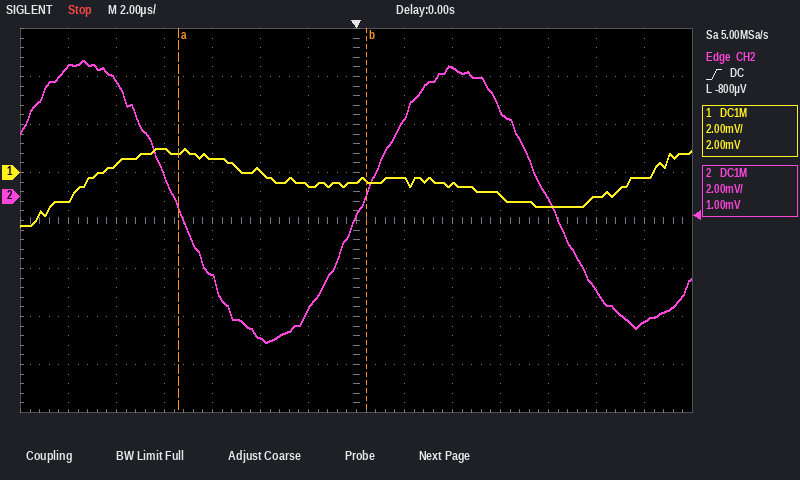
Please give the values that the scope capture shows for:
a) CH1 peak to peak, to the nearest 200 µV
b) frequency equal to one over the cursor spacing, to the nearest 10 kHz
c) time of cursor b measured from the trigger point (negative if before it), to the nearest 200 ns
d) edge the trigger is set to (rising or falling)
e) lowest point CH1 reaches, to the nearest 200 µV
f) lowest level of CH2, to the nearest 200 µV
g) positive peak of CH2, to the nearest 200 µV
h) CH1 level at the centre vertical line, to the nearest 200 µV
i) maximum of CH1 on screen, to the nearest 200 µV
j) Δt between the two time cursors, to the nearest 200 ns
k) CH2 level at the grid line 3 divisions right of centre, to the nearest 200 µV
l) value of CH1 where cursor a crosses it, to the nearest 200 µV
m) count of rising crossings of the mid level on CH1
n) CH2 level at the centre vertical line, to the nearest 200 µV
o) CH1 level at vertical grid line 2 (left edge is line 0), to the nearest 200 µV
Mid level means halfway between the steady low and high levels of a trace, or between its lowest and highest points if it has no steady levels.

3.2 mV
130 kHz
+400 ns
rising
-2.2 mV
-6.0 mV
5.6 mV
-400 µV
1.0 mV
7.8 µs
3.6 mV
800 µV
2
-800 µV
400 µV
